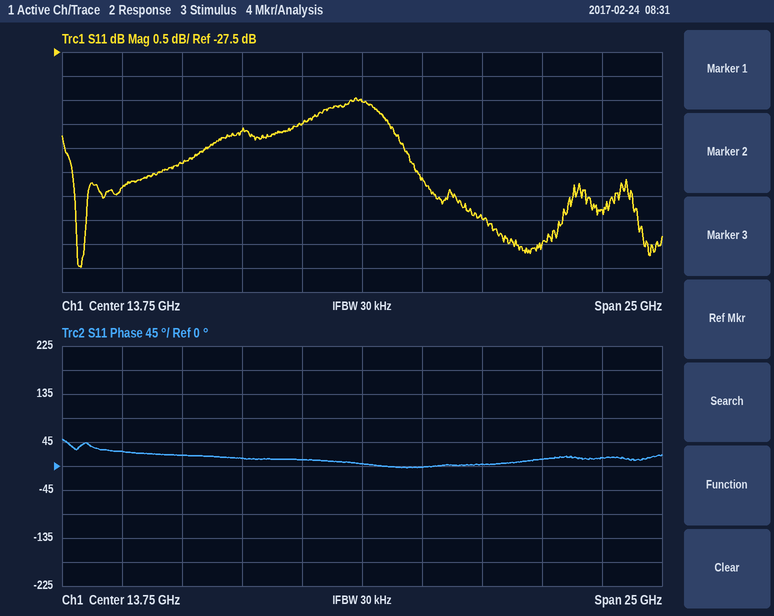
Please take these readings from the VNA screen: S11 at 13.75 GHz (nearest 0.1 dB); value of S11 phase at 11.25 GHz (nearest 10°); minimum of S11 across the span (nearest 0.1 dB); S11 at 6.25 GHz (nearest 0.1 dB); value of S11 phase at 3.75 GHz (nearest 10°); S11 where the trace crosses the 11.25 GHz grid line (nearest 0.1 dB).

-28.5 dB
10°
-32.0 dB
-29.8 dB
30°
-29.0 dB
